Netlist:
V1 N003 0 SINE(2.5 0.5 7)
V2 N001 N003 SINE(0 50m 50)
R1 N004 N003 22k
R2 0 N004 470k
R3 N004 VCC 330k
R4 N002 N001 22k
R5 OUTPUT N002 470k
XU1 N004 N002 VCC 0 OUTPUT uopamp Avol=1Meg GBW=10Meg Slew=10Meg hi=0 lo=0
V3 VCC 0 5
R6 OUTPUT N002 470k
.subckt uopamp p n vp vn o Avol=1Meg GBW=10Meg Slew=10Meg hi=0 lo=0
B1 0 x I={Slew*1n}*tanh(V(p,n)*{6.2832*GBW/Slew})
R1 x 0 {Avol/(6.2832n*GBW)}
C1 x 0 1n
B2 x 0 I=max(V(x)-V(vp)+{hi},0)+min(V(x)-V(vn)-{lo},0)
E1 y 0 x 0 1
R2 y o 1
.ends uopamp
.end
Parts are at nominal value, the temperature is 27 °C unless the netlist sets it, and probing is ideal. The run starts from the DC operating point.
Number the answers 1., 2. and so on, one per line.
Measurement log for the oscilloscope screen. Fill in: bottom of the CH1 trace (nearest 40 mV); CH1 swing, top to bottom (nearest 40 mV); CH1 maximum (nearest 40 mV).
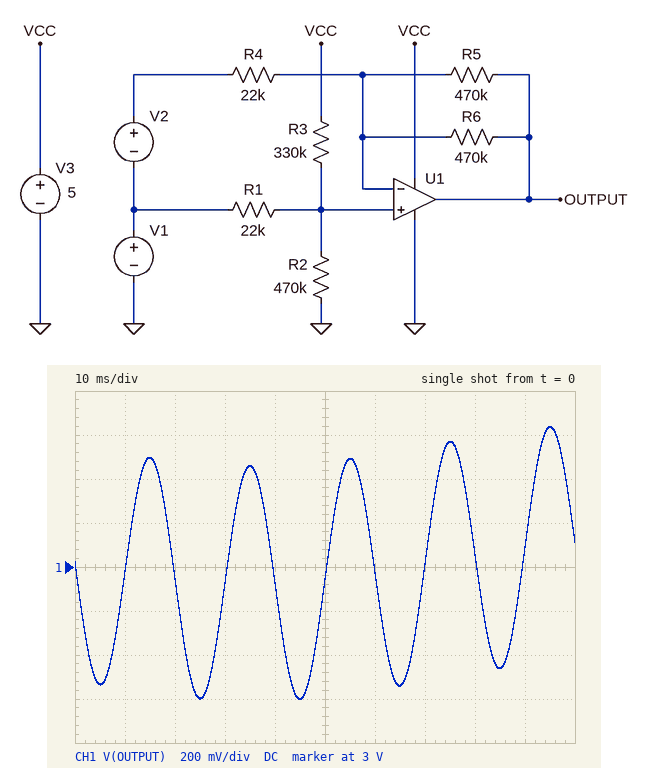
1. 2.40 V
2. 1.24 V
3. 3.64 V
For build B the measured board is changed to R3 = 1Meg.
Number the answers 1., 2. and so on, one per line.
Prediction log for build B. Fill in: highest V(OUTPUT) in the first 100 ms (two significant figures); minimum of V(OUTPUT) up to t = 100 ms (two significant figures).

1. 2.5 V
2. 1.2 V
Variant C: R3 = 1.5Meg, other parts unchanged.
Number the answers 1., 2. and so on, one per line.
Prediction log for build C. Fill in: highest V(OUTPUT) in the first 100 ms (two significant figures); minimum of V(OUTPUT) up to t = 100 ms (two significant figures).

1. 2.3 V
2. 990 mV
